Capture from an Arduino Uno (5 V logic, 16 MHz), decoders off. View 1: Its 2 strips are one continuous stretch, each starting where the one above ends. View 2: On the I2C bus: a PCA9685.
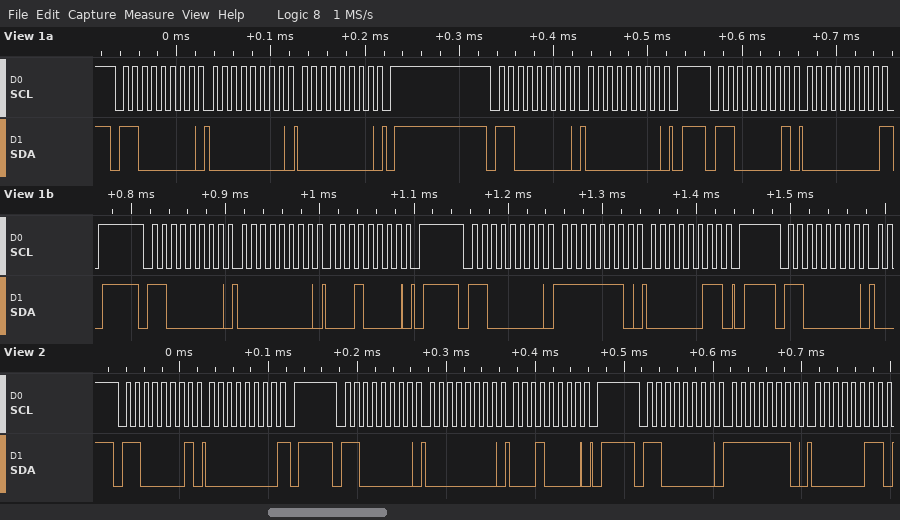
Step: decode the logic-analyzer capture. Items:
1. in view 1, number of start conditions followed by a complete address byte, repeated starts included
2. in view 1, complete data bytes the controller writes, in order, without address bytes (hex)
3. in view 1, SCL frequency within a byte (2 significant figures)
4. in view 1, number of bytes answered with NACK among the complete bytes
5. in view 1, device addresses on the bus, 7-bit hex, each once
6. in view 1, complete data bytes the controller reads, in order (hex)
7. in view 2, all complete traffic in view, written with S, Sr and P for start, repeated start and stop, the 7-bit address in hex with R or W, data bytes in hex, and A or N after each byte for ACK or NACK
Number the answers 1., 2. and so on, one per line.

1. 6
2. 00 00 00 00 10 FE 03
3. 100 kHz
4. 1
5. 0x60
6. 00
7. S 60R A 00 N P S 60W A 00 A 10 A P S 60W A FE A 03 A
